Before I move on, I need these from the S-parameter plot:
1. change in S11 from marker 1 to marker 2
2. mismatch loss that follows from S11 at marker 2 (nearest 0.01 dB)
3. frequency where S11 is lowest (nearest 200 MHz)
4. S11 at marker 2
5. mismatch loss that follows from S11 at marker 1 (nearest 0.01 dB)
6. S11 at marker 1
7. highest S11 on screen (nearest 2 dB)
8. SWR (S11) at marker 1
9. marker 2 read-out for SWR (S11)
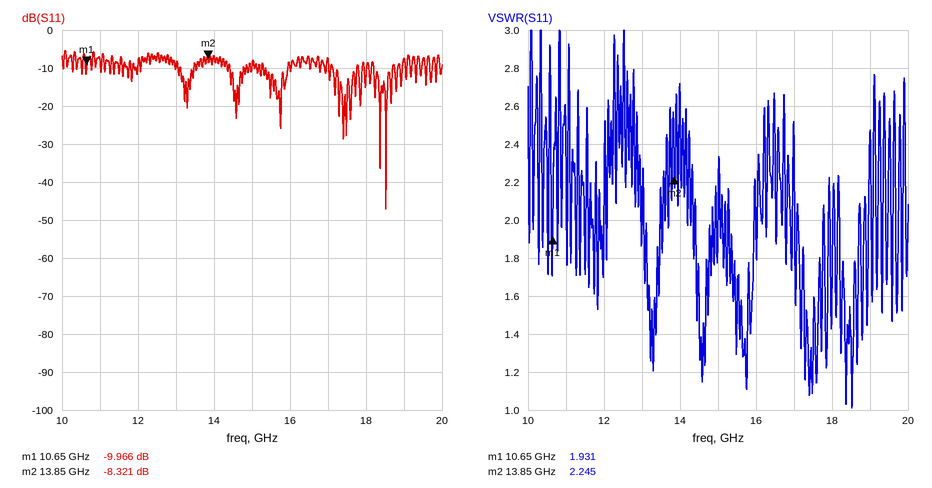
1.645 dB
0.69 dB
18.6 GHz
-8.321 dB
0.46 dB
-9.966 dB
-6 dB
1.931
2.245
